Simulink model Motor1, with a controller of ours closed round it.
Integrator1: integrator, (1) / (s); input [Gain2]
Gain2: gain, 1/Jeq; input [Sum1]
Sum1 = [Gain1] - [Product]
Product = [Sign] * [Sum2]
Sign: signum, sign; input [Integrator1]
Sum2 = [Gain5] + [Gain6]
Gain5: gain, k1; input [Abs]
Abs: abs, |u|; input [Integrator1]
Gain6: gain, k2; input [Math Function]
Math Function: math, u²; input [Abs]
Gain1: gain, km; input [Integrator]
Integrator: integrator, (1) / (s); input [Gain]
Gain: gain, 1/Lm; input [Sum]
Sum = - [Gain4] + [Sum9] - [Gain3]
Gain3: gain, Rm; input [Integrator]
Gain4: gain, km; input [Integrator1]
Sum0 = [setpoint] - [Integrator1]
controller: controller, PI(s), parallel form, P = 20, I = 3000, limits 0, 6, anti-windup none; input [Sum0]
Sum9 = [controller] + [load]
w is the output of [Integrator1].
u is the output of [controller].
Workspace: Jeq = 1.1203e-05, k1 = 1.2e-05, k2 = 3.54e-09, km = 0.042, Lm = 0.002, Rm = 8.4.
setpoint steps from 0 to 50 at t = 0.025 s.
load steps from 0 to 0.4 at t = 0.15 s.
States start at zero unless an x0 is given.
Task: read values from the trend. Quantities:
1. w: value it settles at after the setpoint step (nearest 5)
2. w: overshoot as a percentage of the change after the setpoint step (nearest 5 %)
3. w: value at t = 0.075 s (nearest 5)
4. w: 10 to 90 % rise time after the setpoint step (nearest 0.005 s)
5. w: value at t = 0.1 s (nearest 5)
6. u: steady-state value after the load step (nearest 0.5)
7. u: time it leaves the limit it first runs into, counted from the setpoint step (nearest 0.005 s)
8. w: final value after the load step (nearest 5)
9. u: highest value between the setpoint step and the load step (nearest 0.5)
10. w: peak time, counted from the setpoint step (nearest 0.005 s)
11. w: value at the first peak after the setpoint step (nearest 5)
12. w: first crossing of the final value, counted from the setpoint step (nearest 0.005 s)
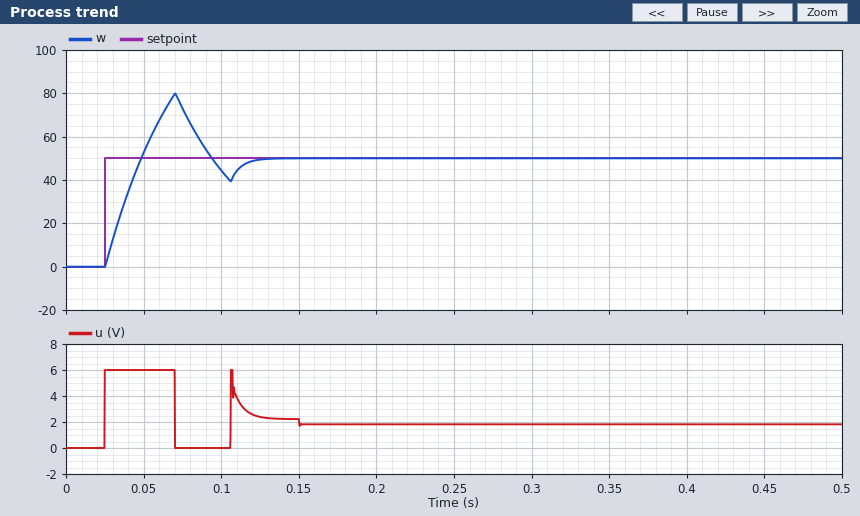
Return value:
50
60 %
75
0.020 s
45
2.0
0.045 s
50
6.0
0.045 s
80
0.025 s
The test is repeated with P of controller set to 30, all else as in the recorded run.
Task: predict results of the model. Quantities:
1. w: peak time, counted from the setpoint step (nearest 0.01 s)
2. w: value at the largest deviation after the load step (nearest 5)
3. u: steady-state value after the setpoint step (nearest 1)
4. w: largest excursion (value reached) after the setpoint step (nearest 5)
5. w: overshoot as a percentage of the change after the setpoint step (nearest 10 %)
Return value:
0.04 s
50
2
75
50 %
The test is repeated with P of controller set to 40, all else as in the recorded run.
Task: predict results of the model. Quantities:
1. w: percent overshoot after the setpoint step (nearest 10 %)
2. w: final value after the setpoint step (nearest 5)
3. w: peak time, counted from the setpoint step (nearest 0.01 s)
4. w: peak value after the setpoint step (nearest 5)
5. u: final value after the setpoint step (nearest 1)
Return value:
50 %
50
0.04 s
75
2
